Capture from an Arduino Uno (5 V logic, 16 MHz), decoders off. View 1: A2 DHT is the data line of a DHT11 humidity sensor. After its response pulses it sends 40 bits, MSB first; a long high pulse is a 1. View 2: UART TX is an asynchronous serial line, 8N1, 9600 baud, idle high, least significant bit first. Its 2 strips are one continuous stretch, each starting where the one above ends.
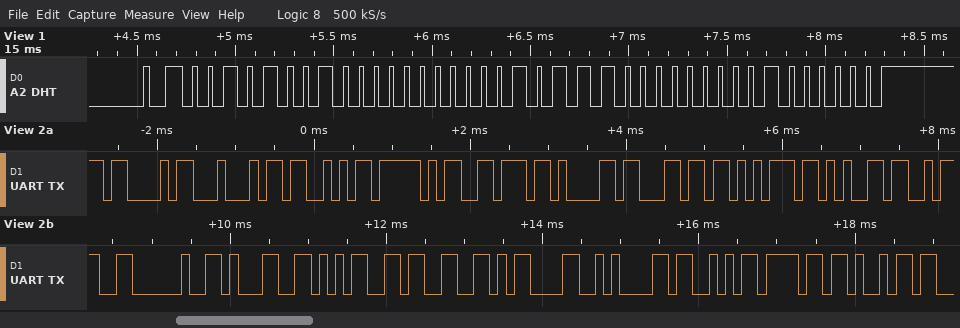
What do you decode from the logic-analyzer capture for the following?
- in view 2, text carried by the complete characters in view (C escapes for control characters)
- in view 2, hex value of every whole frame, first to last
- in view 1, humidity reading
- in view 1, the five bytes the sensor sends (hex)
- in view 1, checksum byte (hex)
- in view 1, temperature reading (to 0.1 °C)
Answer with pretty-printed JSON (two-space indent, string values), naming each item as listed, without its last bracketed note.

{
  "in view 2, text carried by the complete characters in view": "\"CDS_value: 153\\r\\nSoi\"",
  "in view 2, hex value of every whole frame, first to last": "43 44 53 5F 76 61 6C 75 65 3A 20 31 35 33 0D 0A 53 6F 69",
  "in view 1, humidity reading": "41 %",
  "in view 1, the five bytes the sensor sends": "29 00 17 00 40",
  "in view 1, checksum byte": "0x40",
  "in view 1, temperature reading": "23.0 °C"
}
